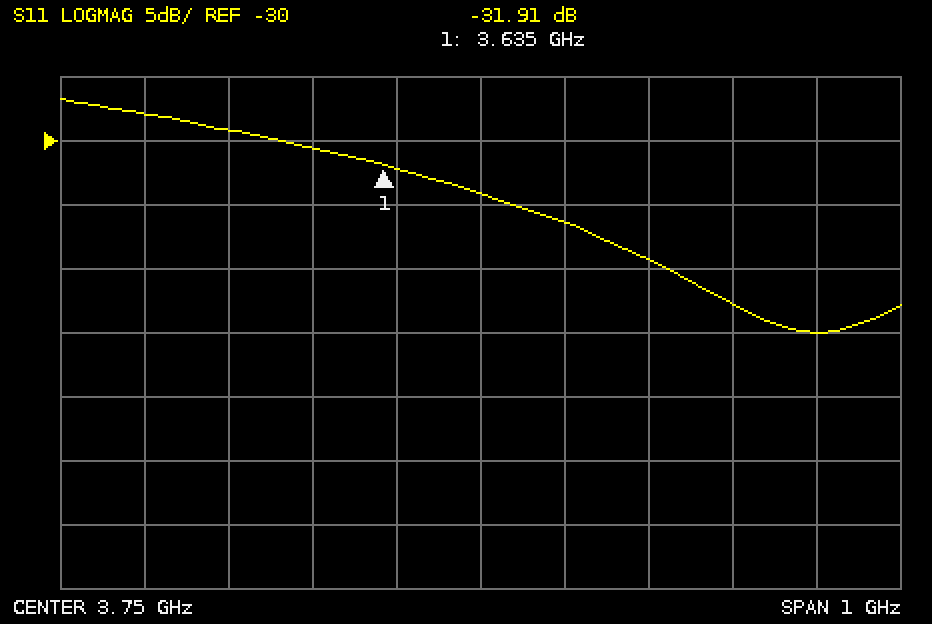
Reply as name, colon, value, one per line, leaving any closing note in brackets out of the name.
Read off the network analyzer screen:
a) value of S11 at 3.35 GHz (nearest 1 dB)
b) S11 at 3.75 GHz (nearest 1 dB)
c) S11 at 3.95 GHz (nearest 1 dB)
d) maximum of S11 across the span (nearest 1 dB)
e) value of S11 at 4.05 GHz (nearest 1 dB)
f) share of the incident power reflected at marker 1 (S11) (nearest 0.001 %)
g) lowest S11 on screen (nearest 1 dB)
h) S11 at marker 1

value of S11 at 3.35 GHz: -28 dB
S11 at 3.75 GHz: -34 dB
S11 at 3.95 GHz: -39 dB
maximum of S11 across the span: -27 dB
value of S11 at 4.05 GHz: -43 dB
share of the incident power reflected at marker 1 (S11): 0.064 %
lowest S11 on screen: -45 dB
S11 at marker 1: -31.91 dB
